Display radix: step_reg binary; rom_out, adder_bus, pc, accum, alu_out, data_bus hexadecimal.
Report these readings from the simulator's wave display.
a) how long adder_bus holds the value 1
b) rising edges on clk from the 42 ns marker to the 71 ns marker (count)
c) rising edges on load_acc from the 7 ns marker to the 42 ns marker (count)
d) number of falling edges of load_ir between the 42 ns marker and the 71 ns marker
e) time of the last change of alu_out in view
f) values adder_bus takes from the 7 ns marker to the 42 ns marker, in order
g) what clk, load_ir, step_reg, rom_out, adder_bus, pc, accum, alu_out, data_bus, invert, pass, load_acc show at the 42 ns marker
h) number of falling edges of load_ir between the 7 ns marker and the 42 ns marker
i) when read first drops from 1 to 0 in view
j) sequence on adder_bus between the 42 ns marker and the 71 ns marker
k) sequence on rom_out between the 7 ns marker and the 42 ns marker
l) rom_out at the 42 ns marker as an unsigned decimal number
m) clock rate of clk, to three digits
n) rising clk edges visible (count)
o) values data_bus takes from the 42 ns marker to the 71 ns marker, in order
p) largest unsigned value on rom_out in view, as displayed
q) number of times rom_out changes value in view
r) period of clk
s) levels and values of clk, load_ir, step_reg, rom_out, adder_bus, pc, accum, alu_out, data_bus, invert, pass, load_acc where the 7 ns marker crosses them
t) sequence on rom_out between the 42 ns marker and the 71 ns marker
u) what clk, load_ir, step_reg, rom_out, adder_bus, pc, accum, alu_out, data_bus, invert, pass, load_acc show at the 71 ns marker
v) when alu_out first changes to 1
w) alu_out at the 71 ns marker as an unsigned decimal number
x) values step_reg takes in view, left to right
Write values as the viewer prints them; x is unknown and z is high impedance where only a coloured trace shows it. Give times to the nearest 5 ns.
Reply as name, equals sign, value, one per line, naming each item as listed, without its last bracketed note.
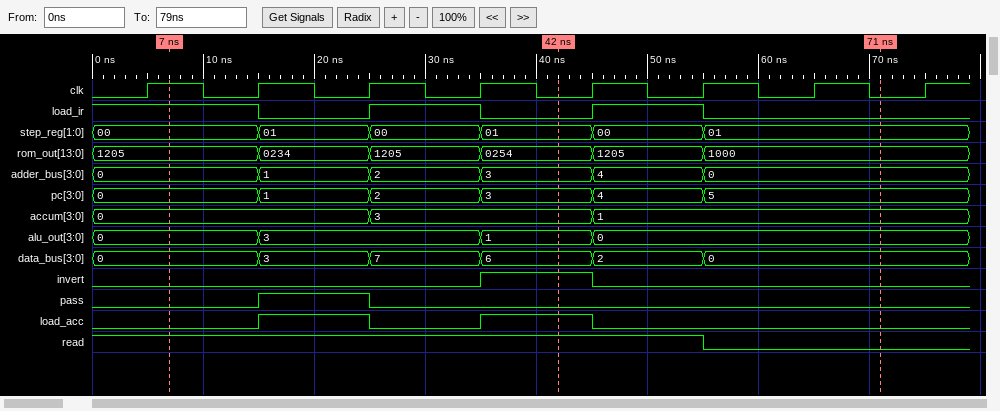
how long adder_bus holds the value 1 = 10 ns
rising edges on clk from the 42 ns marker to the 71 ns marker = 3
rising edges on load_acc from the 7 ns marker to the 42 ns marker = 2
number of falling edges of load_ir between the 42 ns marker and the 71 ns marker = 1
time of the last change of alu_out in view = 45 ns
values adder_bus takes from the 7 ns marker to the 42 ns marker, in order = 0, 1, 2, 3
what clk, load_ir, step_reg, rom_out, adder_bus, pc, accum, alu_out, data_bus, invert, pass, load_acc show at the 42 ns marker = clk=0, load_ir=0, step_reg=01, rom_out=0254, adder_bus=3, pc=3, accum=3, alu_out=1, data_bus=6, invert=1, pass=0, load_acc=1
number of falling edges of load_ir between the 7 ns marker and the 42 ns marker = 2
when read first drops from 1 to 0 in view = 55 ns
sequence on adder_bus between the 42 ns marker and the 71 ns marker = 3, 4, 0
sequence on rom_out between the 7 ns marker and the 42 ns marker = 1205, 0234, 1205, 0254
rom_out at the 42 ns marker as an unsigned decimal number = 596
clock rate of clk, to three digits = 100 MHz
rising clk edges visible = 8
values data_bus takes from the 42 ns marker to the 71 ns marker, in order = 6, 2, 0
largest unsigned value on rom_out in view, as displayed = 1205
number of times rom_out changes value in view = 5
period of clk = 10 ns
levels and values of clk, load_ir, step_reg, rom_out, adder_bus, pc, accum, alu_out, data_bus, invert, pass, load_acc where the 7 ns marker crosses them = clk=1, load_ir=1, step_reg=00, rom_out=1205, adder_bus=0, pc=0, accum=0, alu_out=0, data_bus=0, invert=0, pass=0, load_acc=0
sequence on rom_out between the 42 ns marker and the 71 ns marker = 0254, 1205, 1000
what clk, load_ir, step_reg, rom_out, adder_bus, pc, accum, alu_out, data_bus, invert, pass, load_acc show at the 71 ns marker = clk=0, load_ir=0, step_reg=01, rom_out=1000, adder_bus=0, pc=5, accum=1, alu_out=0, data_bus=0, invert=0, pass=0, load_acc=0
when alu_out first changes to 1 = 35 ns
alu_out at the 71 ns marker as an unsigned decimal number = 0
values step_reg takes in view, left to right = 00, 01, 00, 01, 00, 01
